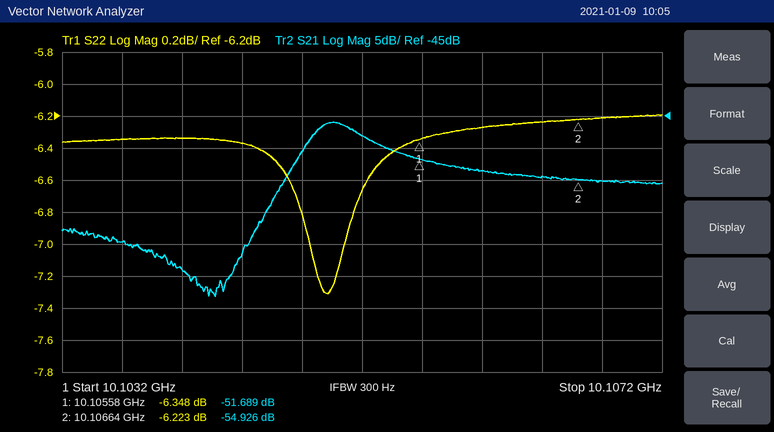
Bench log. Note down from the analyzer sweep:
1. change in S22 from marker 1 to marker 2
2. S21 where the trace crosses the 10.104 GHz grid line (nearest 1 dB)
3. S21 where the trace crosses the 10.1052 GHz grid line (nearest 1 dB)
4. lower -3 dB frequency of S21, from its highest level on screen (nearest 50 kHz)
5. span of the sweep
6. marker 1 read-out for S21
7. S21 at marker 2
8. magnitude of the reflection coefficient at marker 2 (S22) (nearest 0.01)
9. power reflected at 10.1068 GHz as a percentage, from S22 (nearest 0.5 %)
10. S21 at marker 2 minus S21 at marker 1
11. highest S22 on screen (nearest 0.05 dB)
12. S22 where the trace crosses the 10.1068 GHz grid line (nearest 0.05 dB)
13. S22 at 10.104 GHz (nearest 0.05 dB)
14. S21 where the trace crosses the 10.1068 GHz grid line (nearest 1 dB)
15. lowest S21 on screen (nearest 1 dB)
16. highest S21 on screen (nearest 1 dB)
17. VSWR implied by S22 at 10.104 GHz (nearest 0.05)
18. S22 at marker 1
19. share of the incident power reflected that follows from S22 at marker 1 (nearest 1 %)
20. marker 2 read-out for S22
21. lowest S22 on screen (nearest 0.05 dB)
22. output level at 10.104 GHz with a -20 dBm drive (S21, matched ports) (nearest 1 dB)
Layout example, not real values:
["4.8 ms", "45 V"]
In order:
["0.125 dB", "-69 dB", "-48 dB", "10.10485 GHz", "4 MHz", "-51.689 dB", "-54.926 dB", "0.49", "24.0 %", "-3.237 dB", "-6.20 dB", "-6.20 dB", "-6.35 dB", "-55 dB", "-73 dB", "-46 dB", "2.85", "-6.348 dB", "23 %", "-6.223 dB", "-7.30 dB", "-89 dBm"]
